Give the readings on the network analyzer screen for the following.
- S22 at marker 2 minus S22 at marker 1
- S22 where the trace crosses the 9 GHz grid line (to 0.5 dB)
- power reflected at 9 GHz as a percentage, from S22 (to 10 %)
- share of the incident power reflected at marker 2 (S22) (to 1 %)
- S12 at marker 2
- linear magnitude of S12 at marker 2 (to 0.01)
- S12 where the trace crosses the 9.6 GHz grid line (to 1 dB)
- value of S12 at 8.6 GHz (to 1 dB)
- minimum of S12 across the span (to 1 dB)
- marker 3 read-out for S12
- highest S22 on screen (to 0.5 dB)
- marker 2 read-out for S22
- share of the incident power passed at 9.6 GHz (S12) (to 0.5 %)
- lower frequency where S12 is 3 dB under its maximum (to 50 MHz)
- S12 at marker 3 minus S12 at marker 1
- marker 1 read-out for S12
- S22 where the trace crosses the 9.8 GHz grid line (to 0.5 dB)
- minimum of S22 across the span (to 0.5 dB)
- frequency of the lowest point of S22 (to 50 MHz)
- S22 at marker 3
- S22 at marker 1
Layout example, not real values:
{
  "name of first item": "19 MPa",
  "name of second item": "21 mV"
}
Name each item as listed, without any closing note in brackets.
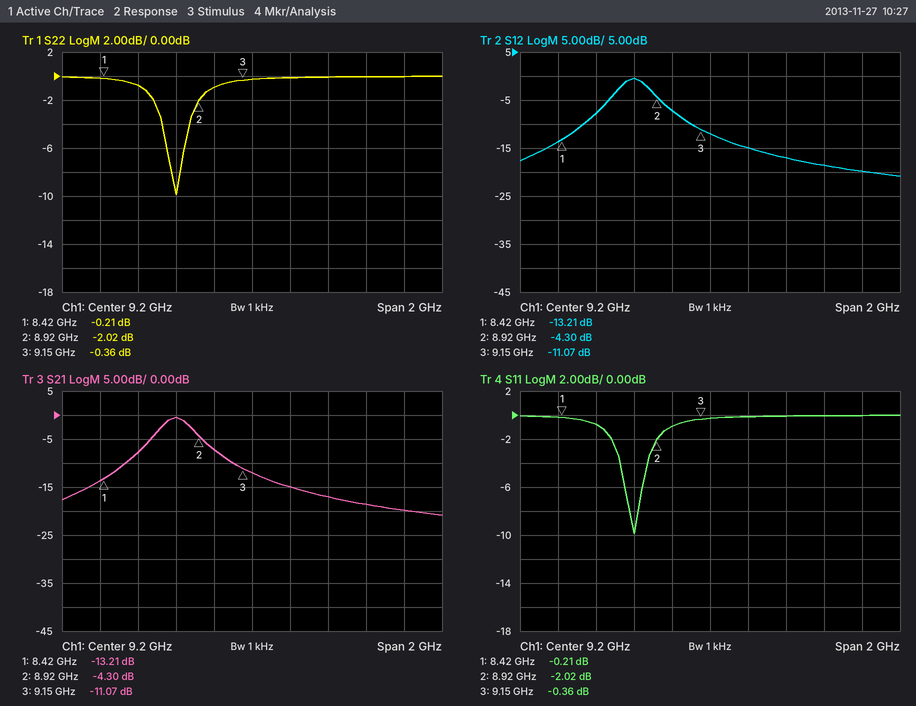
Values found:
{
  "S22 at marker 2 minus S22 at marker 1": "-1.81 dB",
  "S22 where the trace crosses the 9 GHz grid line": "-1.0 dB",
  "power reflected at 9 GHz as a percentage, from S22": "80 %",
  "share of the incident power reflected at marker 2 (S22)": "63 %",
  "S12 at marker 2": "-4.30 dB",
  "linear magnitude of S12 at marker 2": "0.61",
  "S12 where the trace crosses the 9.6 GHz grid line": "-17 dB",
  "value of S12 at 8.6 GHz": "-8 dB",
  "minimum of S12 across the span": "-21 dB",
  "marker 3 read-out for S12": "-11.07 dB",
  "highest S22 on screen": "0.0 dB",
  "marker 2 read-out for S22": "-2.02 dB",
  "share of the incident power passed at 9.6 GHz (S12)": "2.0 %",
  "lower frequency where S12 is 3 dB under its maximum": "8.70 GHz",
  "S12 at marker 3 minus S12 at marker 1": "2.14 dB",
  "marker 1 read-out for S12": "-13.21 dB",
  "S22 where the trace crosses the 9.8 GHz grid line": "0.0 dB",
  "minimum of S22 across the span": "-10.0 dB",
  "frequency of the lowest point of S22": "8.80 GHz",
  "S22 at marker 3": "-0.36 dB",
  "S22 at marker 1": "-0.21 dB"
}
